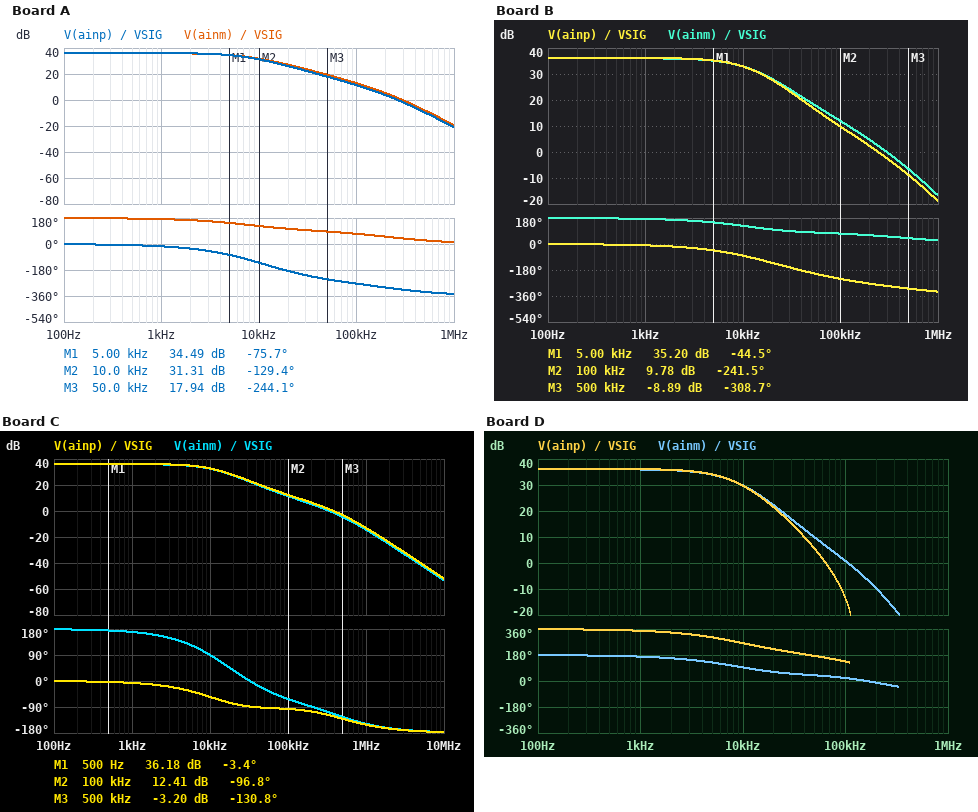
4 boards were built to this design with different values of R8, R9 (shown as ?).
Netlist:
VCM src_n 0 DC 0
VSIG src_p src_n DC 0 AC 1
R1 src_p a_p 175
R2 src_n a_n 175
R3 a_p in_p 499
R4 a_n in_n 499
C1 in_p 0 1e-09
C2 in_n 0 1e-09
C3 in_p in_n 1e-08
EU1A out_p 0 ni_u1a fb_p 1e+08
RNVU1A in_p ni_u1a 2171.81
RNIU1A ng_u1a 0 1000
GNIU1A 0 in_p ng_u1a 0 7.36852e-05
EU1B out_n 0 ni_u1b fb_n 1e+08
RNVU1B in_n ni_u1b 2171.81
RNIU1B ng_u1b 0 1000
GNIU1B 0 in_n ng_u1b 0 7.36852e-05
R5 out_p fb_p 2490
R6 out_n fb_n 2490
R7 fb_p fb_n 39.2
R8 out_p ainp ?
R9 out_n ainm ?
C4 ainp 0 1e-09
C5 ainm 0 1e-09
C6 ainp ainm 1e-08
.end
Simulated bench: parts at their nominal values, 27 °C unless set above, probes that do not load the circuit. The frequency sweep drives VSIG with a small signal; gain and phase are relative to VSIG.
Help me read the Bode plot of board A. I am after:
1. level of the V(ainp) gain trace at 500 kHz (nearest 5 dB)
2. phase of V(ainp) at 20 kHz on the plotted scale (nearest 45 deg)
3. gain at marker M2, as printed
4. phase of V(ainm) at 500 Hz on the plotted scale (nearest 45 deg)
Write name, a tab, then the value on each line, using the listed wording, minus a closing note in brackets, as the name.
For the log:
level of the V(ainp) gain trace at 500 kHz	-10 dB
phase of V(ainp) at 20 kHz on the plotted scale	-180 deg
gain at marker M2, as printed	31.31 dB
phase of V(ainm) at 500 Hz on the plotted scale	180 deg
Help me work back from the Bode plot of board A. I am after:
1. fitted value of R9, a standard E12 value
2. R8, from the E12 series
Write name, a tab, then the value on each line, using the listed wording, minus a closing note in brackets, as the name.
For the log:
fitted value of R9, a standard E12 value	330 Ω
R8, from the E12 series	1.5 kΩ
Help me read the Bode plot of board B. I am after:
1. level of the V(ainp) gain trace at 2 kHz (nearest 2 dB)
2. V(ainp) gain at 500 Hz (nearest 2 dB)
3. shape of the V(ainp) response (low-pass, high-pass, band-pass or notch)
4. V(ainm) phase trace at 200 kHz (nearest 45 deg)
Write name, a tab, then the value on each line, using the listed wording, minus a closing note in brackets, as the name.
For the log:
level of the V(ainp) gain trace at 2 kHz	36 dB
V(ainp) gain at 500 Hz	36 dB
shape of the V(ainp) response	low-pass
V(ainm) phase trace at 200 kHz	45 deg
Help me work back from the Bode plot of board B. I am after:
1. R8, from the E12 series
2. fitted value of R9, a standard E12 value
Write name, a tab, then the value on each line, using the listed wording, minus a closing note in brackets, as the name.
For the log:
R8, from the E12 series	560 Ω
fitted value of R9, a standard E12 value	180 Ω
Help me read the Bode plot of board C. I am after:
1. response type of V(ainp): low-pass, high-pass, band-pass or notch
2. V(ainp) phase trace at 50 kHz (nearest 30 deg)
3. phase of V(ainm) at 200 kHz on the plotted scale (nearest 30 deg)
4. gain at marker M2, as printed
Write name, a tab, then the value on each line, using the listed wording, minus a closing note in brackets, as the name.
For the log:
response type of V(ainp): low-pass, high-pass, band-pass or notch	low-pass
V(ainp) phase trace at 50 kHz	-90 deg
phase of V(ainm) at 200 kHz on the plotted scale	-90 deg
gain at marker M2, as printed	12.41 dB
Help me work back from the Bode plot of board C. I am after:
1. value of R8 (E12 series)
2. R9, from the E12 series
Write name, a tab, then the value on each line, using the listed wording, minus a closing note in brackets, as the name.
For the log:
value of R8	220 Ω
R9, from the E12 series	680 Ω
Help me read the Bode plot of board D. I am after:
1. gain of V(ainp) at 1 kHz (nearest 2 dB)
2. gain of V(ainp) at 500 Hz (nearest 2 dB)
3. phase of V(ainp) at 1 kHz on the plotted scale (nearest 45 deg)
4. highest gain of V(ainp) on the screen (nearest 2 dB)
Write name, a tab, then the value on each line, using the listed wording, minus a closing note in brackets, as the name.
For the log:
gain of V(ainp) at 1 kHz	36 dB
gain of V(ainp) at 500 Hz	36 dB
phase of V(ainp) at 1 kHz on the plotted scale	360 deg
highest gain of V(ainp) on the screen	36 dB
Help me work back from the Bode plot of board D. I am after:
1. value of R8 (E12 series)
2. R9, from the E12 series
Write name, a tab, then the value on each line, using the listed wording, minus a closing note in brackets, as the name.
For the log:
value of R8	1 kΩ
R9, from the E12 series	820 Ω
